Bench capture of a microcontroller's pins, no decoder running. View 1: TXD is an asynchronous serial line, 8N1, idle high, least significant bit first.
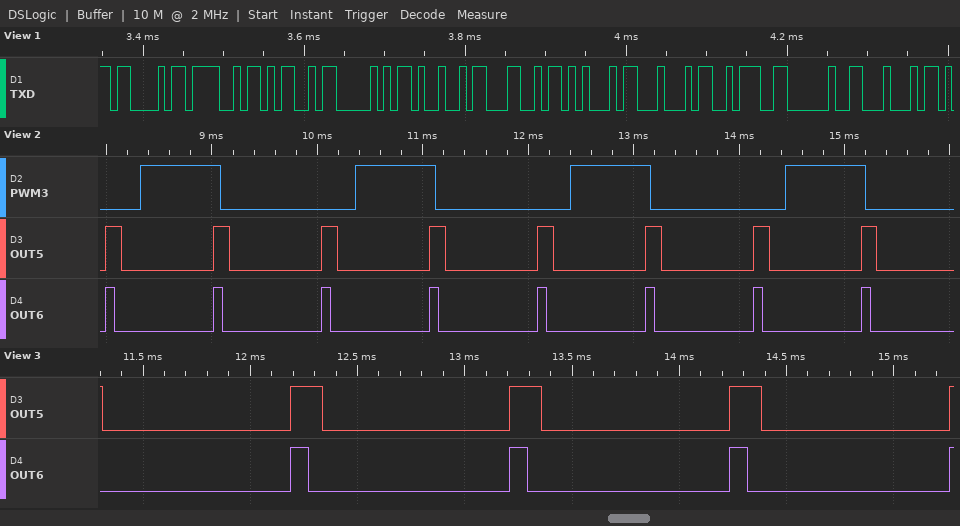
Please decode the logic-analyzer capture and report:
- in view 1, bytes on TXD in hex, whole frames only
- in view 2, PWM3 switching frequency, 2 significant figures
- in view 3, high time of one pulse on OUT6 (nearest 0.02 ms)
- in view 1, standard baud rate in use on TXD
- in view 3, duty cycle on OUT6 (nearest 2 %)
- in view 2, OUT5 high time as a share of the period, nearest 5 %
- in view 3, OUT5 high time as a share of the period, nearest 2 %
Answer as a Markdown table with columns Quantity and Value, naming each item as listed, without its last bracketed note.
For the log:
| Quantity | Value |
|---|---|
| in view 1, bytes on TXD in hex, whole frames only | 43 4F 4D 50 49 4C 45 44 3A 20 44 |
| in view 2, PWM3 switching frequency, 2 significant figures | 490 Hz |
| in view 3, high time of one pulse on OUT6 | 0.08 ms |
| in view 1, standard baud rate in use on TXD | 115200 baud |
| in view 3, duty cycle on OUT6 | 8 % |
| in view 2, OUT5 high time as a share of the period, nearest 5 % | 15 % |
| in view 3, OUT5 high time as a share of the period, nearest 2 % | 14 % |
